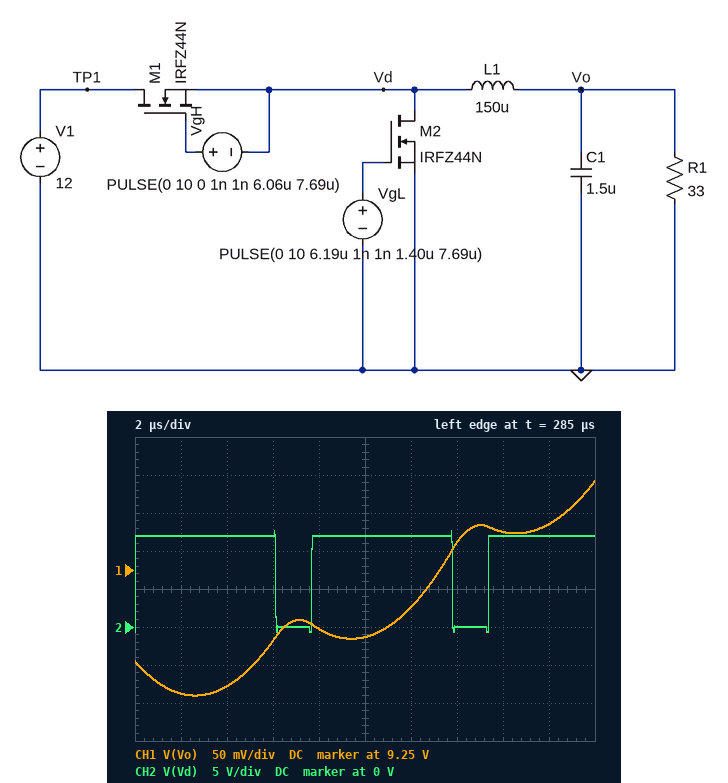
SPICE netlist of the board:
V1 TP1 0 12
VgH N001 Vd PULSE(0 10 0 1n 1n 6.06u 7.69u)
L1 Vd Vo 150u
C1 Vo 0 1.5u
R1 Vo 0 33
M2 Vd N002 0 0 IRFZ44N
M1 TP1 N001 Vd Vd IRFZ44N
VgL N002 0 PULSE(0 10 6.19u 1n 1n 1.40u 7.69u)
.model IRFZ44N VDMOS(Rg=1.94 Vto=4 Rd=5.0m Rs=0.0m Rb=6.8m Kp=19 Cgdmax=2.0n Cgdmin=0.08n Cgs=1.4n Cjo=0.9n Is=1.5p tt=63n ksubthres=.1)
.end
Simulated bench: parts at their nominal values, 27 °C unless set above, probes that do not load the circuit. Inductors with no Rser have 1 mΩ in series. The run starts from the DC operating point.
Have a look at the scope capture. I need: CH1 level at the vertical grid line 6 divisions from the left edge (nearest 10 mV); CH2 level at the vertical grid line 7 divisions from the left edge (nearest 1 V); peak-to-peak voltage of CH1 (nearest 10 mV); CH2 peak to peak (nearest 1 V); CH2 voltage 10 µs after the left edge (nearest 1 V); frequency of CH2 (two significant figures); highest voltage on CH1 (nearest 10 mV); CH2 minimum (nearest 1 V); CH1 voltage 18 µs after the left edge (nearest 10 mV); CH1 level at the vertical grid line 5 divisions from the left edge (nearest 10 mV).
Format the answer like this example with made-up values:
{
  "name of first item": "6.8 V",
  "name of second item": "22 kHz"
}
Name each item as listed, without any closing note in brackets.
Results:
{
  "CH1 level at the vertical grid line 6 divisions from the left edge": "9.20 V",
  "CH2 level at the vertical grid line 7 divisions from the left edge": "0 V",
  "peak-to-peak voltage of CH1": "280 mV",
  "CH2 peak to peak": "13 V",
  "CH2 voltage 10 µs after the left edge": "12 V",
  "frequency of CH2": "130 kHz",
  "highest voltage on CH1": "9.37 V",
  "CH2 minimum": "-1 V",
  "CH1 voltage 18 µs after the left edge": "9.31 V",
  "CH1 level at the vertical grid line 5 divisions from the left edge": "9.16 V"
}
